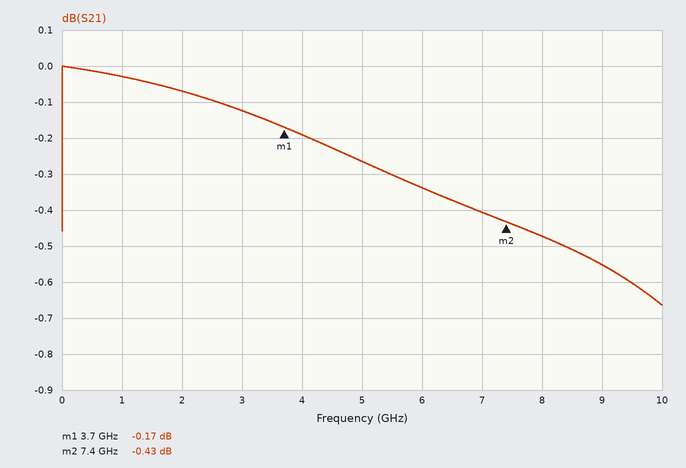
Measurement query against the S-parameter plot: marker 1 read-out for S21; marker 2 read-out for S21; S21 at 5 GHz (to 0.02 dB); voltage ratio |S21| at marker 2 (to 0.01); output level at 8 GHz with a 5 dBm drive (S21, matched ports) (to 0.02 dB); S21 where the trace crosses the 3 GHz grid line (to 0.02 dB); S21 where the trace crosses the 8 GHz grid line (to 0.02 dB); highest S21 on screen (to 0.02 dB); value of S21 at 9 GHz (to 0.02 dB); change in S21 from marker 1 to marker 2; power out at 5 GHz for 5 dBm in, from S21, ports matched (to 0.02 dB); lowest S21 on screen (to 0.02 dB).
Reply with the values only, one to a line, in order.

-0.17 dB
-0.43 dB
-0.26 dB
0.95
4.52 dBm
-0.12 dB
-0.48 dB
0.00 dB
-0.56 dB
-0.26 dB
4.74 dBm
-0.66 dB
